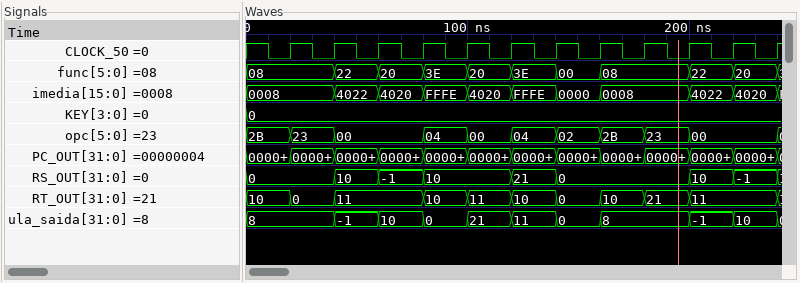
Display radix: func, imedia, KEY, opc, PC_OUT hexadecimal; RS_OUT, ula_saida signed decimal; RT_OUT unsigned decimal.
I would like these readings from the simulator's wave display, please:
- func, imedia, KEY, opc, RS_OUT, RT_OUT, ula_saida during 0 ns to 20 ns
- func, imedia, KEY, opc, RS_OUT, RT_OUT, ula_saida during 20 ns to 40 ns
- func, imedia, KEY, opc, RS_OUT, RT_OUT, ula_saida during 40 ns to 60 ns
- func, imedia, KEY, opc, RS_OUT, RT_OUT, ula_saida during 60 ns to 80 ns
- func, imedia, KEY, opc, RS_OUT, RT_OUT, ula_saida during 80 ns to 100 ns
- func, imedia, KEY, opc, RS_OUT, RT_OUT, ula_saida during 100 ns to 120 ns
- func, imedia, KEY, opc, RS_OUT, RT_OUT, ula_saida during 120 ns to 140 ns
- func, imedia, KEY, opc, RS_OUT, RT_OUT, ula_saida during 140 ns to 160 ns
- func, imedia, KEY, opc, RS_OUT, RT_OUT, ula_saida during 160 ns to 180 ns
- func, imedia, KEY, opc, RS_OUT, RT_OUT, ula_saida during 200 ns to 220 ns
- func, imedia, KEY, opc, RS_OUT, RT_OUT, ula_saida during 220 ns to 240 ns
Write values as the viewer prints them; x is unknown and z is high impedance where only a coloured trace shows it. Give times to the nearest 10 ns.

func=08, imedia=0008, KEY=0, opc=2B, RS_OUT=0, RT_OUT=10, ula_saida=8
func=08, imedia=0008, KEY=0, opc=23, RS_OUT=0, RT_OUT=0, ula_saida=8
func=22, imedia=4022, KEY=0, opc=00, RS_OUT=10, RT_OUT=11, ula_saida=-1
func=20, imedia=4020, KEY=0, opc=00, RS_OUT=-1, RT_OUT=11, ula_saida=10
func=3E, imedia=FFFE, KEY=0, opc=04, RS_OUT=10, RT_OUT=10, ula_saida=0
func=20, imedia=4020, KEY=0, opc=00, RS_OUT=10, RT_OUT=11, ula_saida=21
func=3E, imedia=FFFE, KEY=0, opc=04, RS_OUT=21, RT_OUT=10, ula_saida=11
func=00, imedia=0000, KEY=0, opc=02, RS_OUT=0, RT_OUT=0, ula_saida=0
func=08, imedia=0008, KEY=0, opc=2B, RS_OUT=0, RT_OUT=10, ula_saida=8
func=22, imedia=4022, KEY=0, opc=00, RS_OUT=10, RT_OUT=11, ula_saida=-1
func=20, imedia=4020, KEY=0, opc=00, RS_OUT=-1, RT_OUT=11, ula_saida=10
